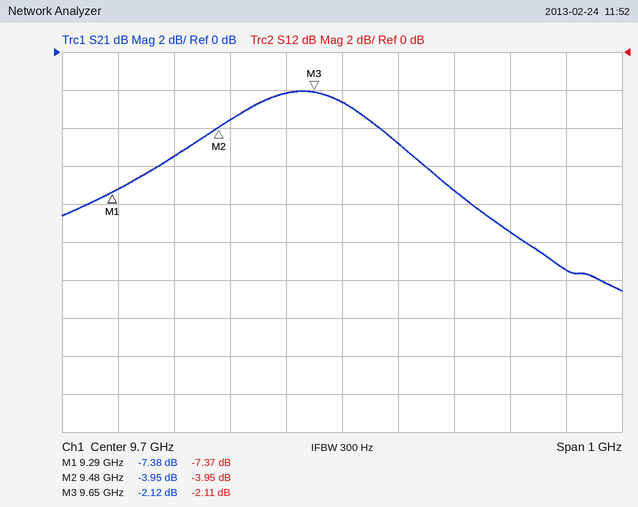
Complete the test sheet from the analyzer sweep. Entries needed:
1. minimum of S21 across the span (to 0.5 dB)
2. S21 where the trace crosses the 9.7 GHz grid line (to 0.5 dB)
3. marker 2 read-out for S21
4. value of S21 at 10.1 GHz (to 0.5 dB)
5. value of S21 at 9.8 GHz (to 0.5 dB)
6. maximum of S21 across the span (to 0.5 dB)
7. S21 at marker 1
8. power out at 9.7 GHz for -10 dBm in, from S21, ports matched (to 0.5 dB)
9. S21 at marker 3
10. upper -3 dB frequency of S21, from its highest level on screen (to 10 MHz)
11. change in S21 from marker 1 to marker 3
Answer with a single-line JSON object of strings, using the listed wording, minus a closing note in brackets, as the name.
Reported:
{"minimum of S21 across the span": "-12.5 dB", "S21 where the trace crosses the 9.7 GHz grid line": "-2.5 dB", "marker 2 read-out for S21": "-3.95 dB", "value of S21 at 10.1 GHz": "-11.5 dB", "value of S21 at 9.8 GHz": "-5.0 dB", "maximum of S21 across the span": "-2.0 dB", "S21 at marker 1": "-7.38 dB", "power out at 9.7 GHz for -10 dBm in, from S21, ports matched": "-12.5 dBm", "S21 at marker 3": "-2.12 dB", "upper -3 dB frequency of S21, from its highest level on screen": "9.81 GHz", "change in S21 from marker 1 to marker 3": "5.26 dB"}
